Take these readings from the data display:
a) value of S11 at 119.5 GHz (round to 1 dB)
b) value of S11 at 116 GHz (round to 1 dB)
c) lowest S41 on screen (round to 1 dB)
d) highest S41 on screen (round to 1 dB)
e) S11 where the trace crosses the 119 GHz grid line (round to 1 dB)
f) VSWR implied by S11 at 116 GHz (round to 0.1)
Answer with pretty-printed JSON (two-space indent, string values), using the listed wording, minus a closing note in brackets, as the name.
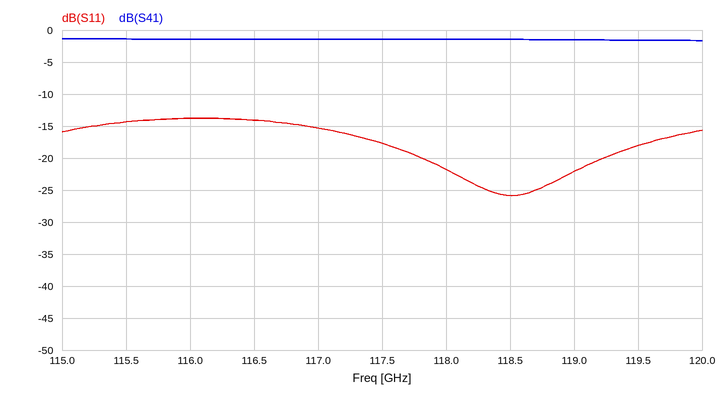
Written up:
{
  "value of S11 at 119.5 GHz": "-18 dB",
  "value of S11 at 116 GHz": "-14 dB",
  "lowest S41 on screen": "-2 dB",
  "highest S41 on screen": "-1 dB",
  "S11 where the trace crosses the 119 GHz grid line": "-22 dB",
  "VSWR implied by S11 at 116 GHz": "1.5"
}
